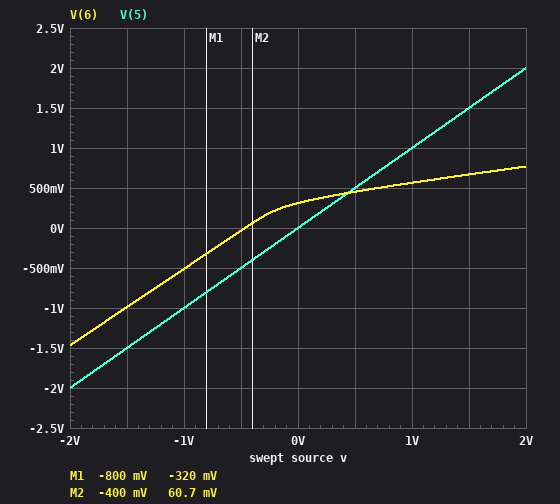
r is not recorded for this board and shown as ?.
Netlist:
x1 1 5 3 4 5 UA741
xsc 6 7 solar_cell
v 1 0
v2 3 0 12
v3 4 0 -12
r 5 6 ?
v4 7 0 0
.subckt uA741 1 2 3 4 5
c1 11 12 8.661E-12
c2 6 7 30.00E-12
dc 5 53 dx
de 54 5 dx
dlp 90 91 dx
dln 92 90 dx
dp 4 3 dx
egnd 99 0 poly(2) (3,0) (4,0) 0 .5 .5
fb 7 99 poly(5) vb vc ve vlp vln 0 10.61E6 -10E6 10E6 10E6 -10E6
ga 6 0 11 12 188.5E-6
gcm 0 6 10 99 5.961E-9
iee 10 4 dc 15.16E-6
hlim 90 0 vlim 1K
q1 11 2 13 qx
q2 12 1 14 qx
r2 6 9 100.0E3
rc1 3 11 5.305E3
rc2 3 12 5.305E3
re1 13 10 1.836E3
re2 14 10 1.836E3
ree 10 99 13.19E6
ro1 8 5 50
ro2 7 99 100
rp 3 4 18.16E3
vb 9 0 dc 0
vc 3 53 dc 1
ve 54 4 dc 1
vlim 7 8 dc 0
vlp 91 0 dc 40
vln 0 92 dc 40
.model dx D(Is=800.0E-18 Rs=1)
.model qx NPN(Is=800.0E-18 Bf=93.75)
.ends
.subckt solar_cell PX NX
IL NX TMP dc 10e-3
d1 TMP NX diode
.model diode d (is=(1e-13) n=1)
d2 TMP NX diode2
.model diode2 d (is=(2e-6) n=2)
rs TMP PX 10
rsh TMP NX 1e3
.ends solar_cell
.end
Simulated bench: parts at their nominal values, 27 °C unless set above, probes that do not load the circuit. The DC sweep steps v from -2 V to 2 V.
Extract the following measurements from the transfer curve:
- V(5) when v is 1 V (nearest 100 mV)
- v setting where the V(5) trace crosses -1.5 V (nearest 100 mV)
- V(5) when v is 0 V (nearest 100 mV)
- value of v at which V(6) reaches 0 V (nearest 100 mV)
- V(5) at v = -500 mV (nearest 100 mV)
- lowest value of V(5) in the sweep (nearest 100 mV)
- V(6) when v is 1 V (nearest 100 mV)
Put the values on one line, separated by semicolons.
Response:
1.0 V; -1.5 V; 0 V; -500 mV; -500 mV; -2.0 V; 600 mV
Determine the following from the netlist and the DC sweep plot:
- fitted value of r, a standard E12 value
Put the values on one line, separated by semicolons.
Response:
47 Ω
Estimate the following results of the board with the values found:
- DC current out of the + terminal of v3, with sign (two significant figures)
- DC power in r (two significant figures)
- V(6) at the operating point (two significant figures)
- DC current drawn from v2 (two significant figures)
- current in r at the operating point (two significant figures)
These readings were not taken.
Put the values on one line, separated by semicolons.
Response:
-1.3 mA; 2.1 mW; 310 mV; 1.3 mA; 6.6 mA
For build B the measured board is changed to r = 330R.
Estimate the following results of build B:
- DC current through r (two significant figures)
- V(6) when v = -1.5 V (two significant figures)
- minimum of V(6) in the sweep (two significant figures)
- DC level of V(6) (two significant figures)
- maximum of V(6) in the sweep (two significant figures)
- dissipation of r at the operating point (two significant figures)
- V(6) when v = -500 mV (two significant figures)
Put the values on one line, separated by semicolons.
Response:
1.3 mA; 340 mV; 300 mV; 420 mV; 500 mV; 530 µW; 390 mV
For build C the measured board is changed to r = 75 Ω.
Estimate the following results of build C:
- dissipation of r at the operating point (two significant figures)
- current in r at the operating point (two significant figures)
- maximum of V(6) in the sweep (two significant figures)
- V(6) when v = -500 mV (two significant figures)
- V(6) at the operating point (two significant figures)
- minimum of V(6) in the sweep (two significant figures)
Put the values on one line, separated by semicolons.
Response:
1.7 mW; 4.7 mA; 670 mV; 190 mV; 360 mV; -1.2 V
